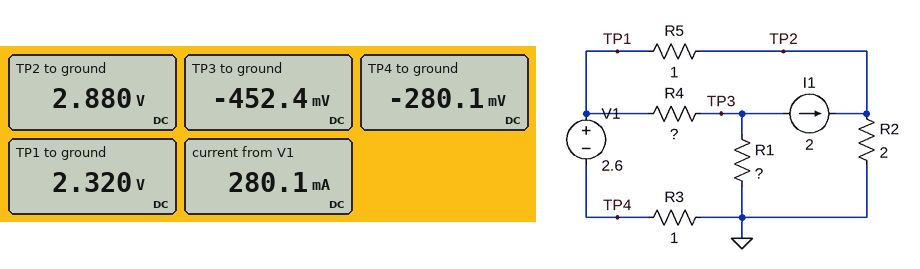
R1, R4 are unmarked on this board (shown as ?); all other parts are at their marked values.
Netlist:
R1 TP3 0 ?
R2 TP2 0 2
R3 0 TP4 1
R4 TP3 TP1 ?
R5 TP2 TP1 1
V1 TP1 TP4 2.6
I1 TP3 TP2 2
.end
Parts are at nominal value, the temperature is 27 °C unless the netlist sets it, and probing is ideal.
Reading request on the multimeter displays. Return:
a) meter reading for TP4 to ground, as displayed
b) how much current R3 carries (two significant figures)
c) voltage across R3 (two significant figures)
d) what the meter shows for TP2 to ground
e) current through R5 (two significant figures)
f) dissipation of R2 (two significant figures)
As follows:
-280.1 mV
280 mA
280 mV
2.880 V
560 mA
4.1 W
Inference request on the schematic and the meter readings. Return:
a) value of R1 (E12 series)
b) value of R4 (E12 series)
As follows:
0.39 Ω
3.3 Ω
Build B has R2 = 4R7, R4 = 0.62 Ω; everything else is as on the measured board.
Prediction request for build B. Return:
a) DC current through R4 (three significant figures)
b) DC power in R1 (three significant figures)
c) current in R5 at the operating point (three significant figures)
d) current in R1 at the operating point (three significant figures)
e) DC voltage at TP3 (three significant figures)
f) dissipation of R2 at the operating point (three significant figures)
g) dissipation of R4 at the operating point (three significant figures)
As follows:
2.36 A
51.1 mW
1.37 A
362 mA
141 mV
1.88 W
3.46 W
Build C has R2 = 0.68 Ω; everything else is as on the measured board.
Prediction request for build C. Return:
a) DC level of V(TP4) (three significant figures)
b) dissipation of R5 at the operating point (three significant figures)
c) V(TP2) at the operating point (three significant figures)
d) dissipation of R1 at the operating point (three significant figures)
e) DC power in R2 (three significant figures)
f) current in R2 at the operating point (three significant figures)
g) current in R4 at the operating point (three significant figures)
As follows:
-886 mV
44.3 mW
1.50 V
684 mW
3.32 W
2.21 A
676 mA
